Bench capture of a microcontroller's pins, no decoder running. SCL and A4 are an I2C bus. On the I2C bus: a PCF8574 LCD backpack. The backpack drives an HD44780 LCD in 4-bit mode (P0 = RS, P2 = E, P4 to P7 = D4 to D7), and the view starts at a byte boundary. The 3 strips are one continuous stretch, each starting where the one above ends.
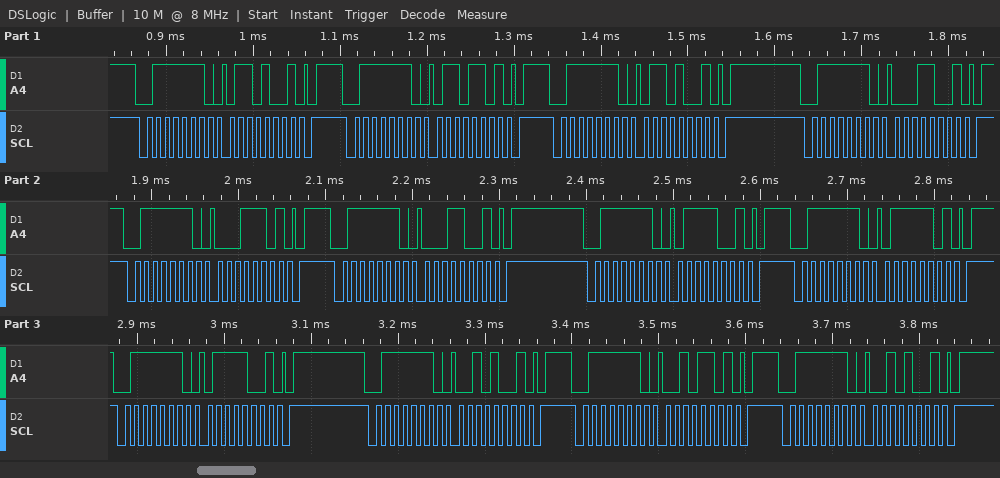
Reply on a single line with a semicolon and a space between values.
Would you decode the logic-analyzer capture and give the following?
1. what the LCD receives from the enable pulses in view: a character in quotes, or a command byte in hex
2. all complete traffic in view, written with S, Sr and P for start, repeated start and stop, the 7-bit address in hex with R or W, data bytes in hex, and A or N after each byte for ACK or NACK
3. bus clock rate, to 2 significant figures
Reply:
'a' 'r'; S 3FW A 69 A P S 3FW A 6D A P S 3FW A 69 A P S 3FW A 19 A P S 3FW A 1D A P S 3FW A 19 A P S 3FW A 79 A P S 3FW A 7D A P S 3FW A 79 A P S 3FW A 29 A P S 3FW A 2D A P S 3FW A 29 A P; 100 kHz
